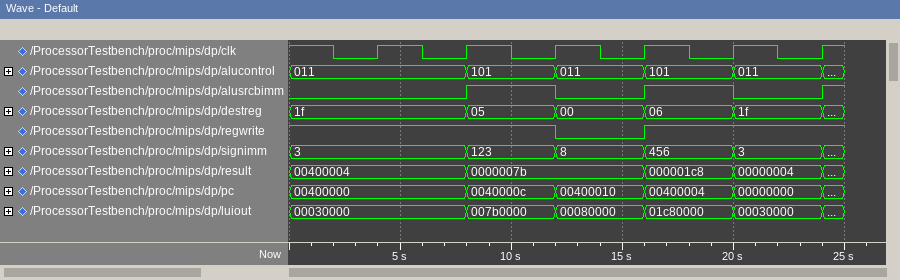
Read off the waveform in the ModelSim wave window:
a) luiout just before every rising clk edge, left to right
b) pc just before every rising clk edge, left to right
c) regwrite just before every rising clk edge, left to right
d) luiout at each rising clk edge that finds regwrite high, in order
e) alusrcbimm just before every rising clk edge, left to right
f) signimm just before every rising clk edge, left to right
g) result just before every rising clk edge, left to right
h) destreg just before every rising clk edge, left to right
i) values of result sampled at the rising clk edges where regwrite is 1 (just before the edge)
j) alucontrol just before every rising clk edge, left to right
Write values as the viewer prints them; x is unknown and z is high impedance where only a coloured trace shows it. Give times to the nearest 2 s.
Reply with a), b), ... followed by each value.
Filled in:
a) 00030000, 00030000, 007b0000, 00080000, 01c80000, 00030000
b) 00400000, 00400000, 0040000c, 00400010, 00400004, 00000000
c) 1 1 1 0 1 1
d) 00030000, 00030000, 007b0000, 01c80000, 00030000
e) 0 0 1 0 1 0
f) 3, 3, 123, 8, 456, 3
g) 00400004, 00400004, 0000007b, 0000007b, 000001c8, 00000004
h) 1f, 1f, 05, 00, 06, 1f
i) 00400004, 00400004, 0000007b, 000001c8, 00000004
j) 011, 011, 101, 011, 101, 011
